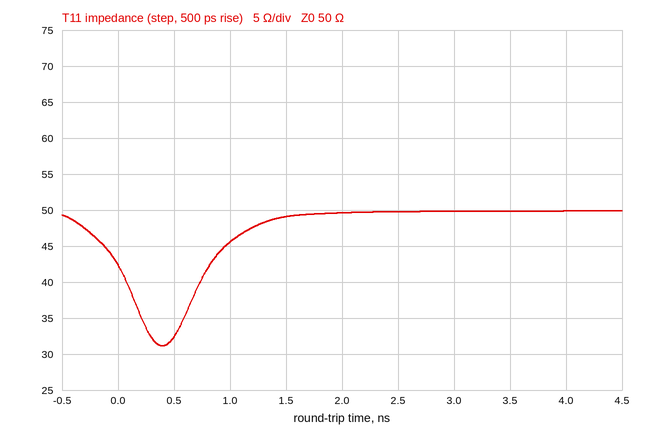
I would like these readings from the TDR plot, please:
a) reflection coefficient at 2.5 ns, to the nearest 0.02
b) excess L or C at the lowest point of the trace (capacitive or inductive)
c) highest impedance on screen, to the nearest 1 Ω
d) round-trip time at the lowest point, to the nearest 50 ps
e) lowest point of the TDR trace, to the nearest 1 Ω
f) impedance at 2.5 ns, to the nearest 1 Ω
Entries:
0.00
capacitive
50 Ω
400 ps
31 Ω
50 Ω
